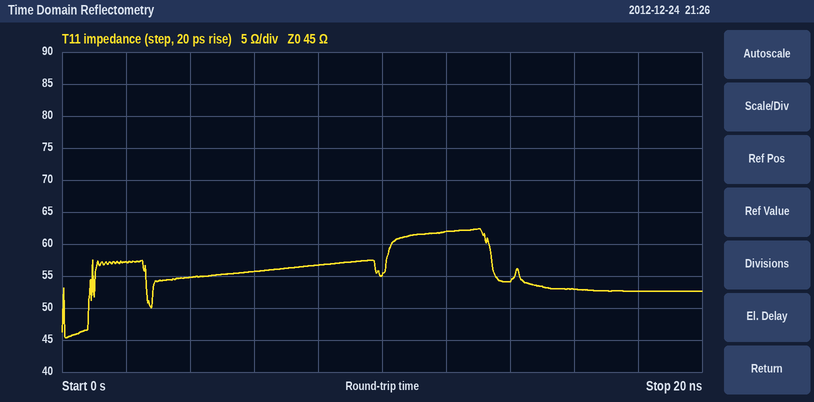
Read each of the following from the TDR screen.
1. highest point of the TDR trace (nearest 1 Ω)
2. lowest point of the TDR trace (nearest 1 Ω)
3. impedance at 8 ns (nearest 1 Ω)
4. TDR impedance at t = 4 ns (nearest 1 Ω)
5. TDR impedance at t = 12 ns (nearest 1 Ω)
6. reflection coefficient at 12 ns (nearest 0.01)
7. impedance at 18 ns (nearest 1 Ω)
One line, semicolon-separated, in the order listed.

62 Ω; 45 Ω; 57 Ω; 55 Ω; 62 Ω; +0.16; 53 Ω
